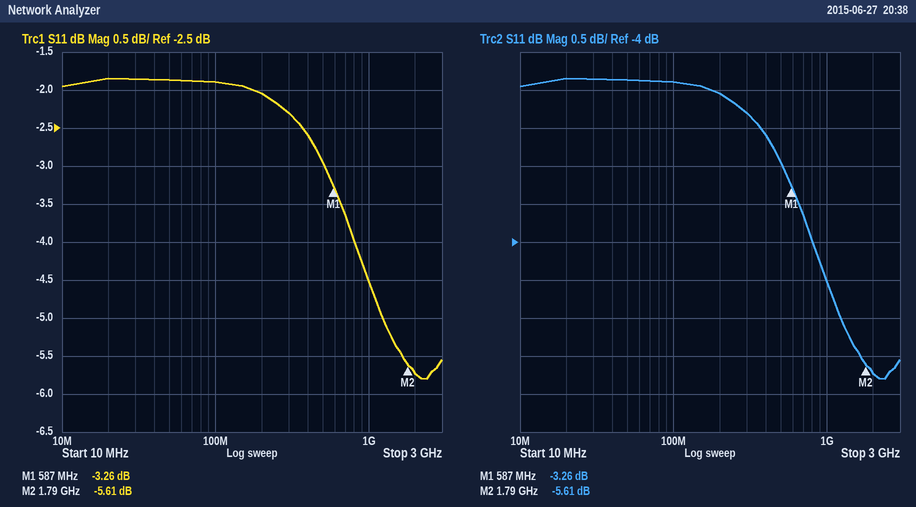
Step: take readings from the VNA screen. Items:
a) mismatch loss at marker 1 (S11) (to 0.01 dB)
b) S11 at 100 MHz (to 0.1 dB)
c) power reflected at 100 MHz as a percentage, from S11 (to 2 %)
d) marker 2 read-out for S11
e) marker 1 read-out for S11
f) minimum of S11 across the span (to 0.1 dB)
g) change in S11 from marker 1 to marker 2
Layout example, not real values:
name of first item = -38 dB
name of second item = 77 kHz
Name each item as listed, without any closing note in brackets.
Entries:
mismatch loss at marker 1 (S11) = 2.77 dB
S11 at 100 MHz = -1.9 dB
power reflected at 100 MHz as a percentage, from S11 = 64 %
marker 2 read-out for S11 = -5.61 dB
marker 1 read-out for S11 = -3.26 dB
minimum of S11 across the span = -5.8 dB
change in S11 from marker 1 to marker 2 = -2.35 dB
